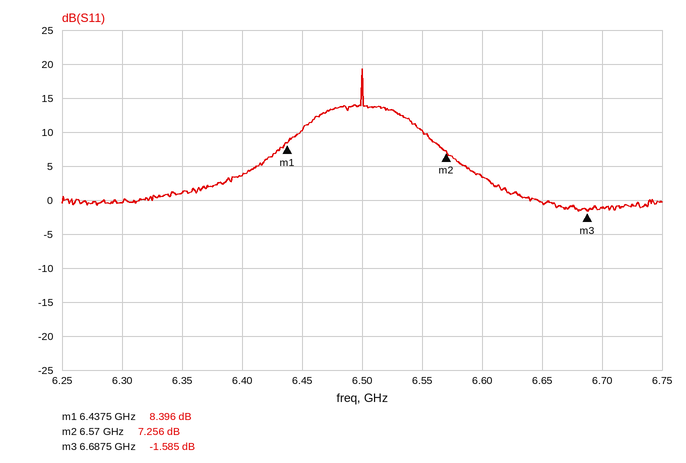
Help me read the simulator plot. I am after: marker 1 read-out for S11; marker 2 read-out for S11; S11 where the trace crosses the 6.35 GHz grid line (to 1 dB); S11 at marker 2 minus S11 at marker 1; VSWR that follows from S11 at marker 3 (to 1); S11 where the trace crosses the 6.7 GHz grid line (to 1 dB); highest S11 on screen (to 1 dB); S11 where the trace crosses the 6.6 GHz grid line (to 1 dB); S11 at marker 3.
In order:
8.396 dB
7.256 dB
1 dB
-1.140 dB
11
-1 dB
19 dB
3 dB
-1.585 dB
